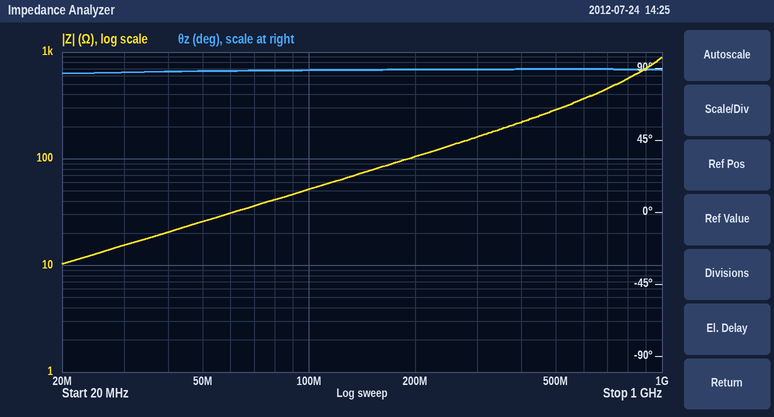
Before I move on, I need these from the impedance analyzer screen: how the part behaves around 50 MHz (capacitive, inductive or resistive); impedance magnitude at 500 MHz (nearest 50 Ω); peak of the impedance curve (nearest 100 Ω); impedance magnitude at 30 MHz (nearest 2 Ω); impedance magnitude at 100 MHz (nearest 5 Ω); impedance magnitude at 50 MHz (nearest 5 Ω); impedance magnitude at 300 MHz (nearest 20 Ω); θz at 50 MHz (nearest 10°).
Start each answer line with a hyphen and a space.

- inductive
- 300 Ω
- 900 Ω
- 16 Ω
- 50 Ω
- 25 Ω
- 160 Ω
- 90°
